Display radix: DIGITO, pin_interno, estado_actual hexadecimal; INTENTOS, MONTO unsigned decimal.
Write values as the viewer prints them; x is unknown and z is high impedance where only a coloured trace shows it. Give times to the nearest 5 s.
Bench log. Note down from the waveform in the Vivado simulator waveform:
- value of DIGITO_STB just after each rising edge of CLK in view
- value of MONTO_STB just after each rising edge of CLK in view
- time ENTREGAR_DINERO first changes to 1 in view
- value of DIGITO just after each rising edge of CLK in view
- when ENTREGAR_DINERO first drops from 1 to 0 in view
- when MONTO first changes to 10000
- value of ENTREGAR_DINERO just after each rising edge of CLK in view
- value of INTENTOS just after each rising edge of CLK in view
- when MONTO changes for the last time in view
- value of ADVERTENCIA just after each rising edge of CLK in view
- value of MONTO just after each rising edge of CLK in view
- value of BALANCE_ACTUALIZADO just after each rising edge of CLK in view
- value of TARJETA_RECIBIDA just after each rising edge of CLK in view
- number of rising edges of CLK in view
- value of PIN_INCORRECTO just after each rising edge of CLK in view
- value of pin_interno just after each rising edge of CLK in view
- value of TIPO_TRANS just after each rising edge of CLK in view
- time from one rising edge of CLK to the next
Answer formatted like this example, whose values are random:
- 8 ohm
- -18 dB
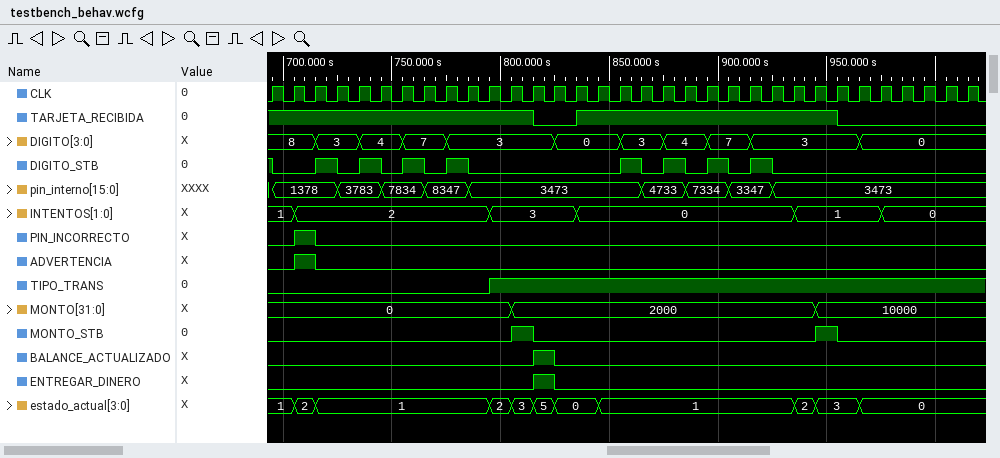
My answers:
- 0 0 1 0 1 0 1 0 1 0 0 0 0 0 0 0 1 0 1 0 1 0 1 0 0 0 0 0 0 0 0 0 0
- 0 0 0 0 0 0 0 0 0 0 0 1 0 0 0 0 0 0 0 0 0 0 0 0 0 1 0 0 0 0 0 0 0
- 815 s
- 8, 8, 3, 3, 4, 4, 7, 7, 3, 3, 3, 3, 3, 0, 0, 0, 3, 3, 4, 4, 7, 7, 3, 3, 3, 3, 3, 0, 0, 0, 0, 0, 0
- 825 s
- 945 s
- 0 0 0 0 0 0 0 0 0 0 0 0 1 0 0 0 0 0 0 0 0 0 0 0 0 0 0 0 0 0 0 0 0
- 1, 2, 2, 2, 2, 2, 2, 2, 2, 2, 3, 3, 3, 3, 0, 0, 0, 0, 0, 0, 0, 0, 0, 0, 1, 1, 1, 1, 0, 0, 0, 0, 0
- 945 s
- 0 1 0 0 0 0 0 0 0 0 0 0 0 0 0 0 0 0 0 0 0 0 0 0 0 0 0 0 0 0 0 0 0
- 0, 0, 0, 0, 0, 0, 0, 0, 0, 0, 0, 2000, 2000, 2000, 2000, 2000, 2000, 2000, 2000, 2000, 2000, 2000, 2000, 2000, 2000, 10000, 10000, 10000, 10000, 10000, 10000, 10000, 10000
- 0 0 0 0 0 0 0 0 0 0 0 0 1 0 0 0 0 0 0 0 0 0 0 0 0 0 0 0 0 0 0 0 0
- 1 1 1 1 1 1 1 1 1 1 1 1 0 0 1 1 1 1 1 1 1 1 1 1 1 1 0 0 0 0 0 0 0
- 33
- 0 1 0 0 0 0 0 0 0 0 0 0 0 0 0 0 0 0 0 0 0 0 0 0 0 0 0 0 0 0 0 0 0
- 1378, 1378, 1378, 3783, 3783, 7834, 7834, 8347, 8347, 3473, 3473, 3473, 3473, 3473, 3473, 3473, 3473, 4733, 4733, 7334, 7334, 3347, 3347, 3473, 3473, 3473, 3473, 3473, 3473, 3473, 3473, 3473, 3473
- 0 0 0 0 0 0 0 0 0 0 1 1 1 1 1 1 1 1 1 1 1 1 1 1 1 1 1 1 1 1 1 1 1
- 10 s
